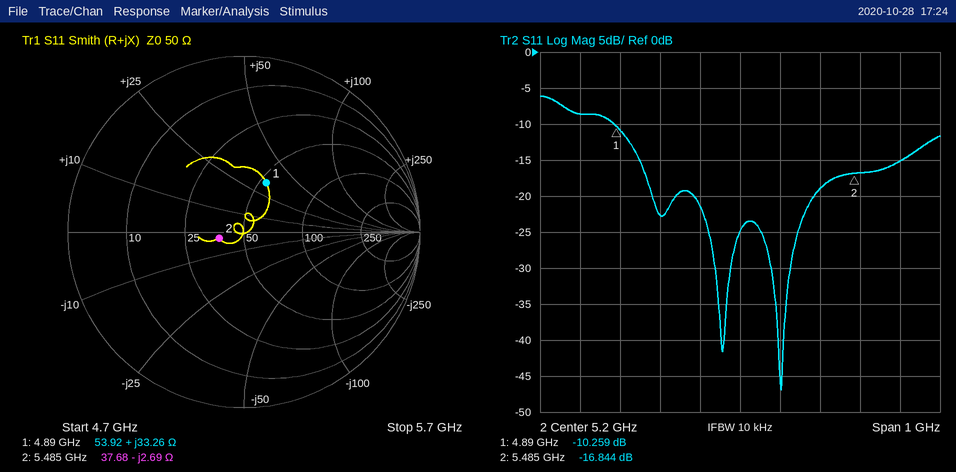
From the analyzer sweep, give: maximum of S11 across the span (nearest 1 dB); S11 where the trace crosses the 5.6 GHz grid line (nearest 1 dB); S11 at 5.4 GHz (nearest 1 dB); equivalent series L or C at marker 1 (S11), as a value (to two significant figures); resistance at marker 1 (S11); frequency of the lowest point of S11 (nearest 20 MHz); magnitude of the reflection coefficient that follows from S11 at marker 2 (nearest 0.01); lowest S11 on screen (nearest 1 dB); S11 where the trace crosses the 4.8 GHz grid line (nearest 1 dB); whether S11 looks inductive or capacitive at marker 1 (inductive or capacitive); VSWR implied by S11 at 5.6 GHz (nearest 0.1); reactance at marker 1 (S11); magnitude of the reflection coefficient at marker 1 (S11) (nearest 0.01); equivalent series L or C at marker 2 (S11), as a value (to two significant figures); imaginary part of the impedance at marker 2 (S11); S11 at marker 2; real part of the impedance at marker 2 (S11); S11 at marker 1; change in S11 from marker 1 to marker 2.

-6 dB
-15 dB
-19 dB
1.1 nH
53.92 Ω
5.30 GHz
0.14
-47 dB
-9 dB
inductive
1.4
+33.26 Ω
0.31
11 pF
-2.69 Ω
-16.844 dB
37.68 Ω
-10.259 dB
-6.585 dB
